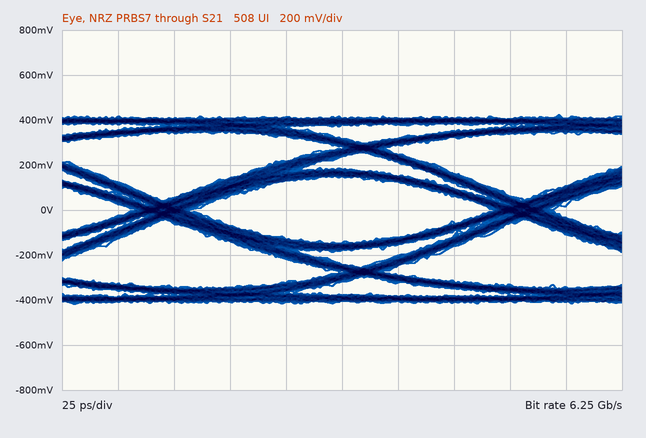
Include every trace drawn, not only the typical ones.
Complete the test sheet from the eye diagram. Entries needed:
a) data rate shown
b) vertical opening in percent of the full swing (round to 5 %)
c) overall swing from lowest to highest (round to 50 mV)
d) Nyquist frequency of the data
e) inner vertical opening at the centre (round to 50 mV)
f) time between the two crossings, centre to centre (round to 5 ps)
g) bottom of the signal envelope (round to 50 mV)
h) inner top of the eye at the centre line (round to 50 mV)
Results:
6.25 Gb/s
35 %
850 mV
3.125 GHz
300 mV
160 ps
-400 mV
150 mV
